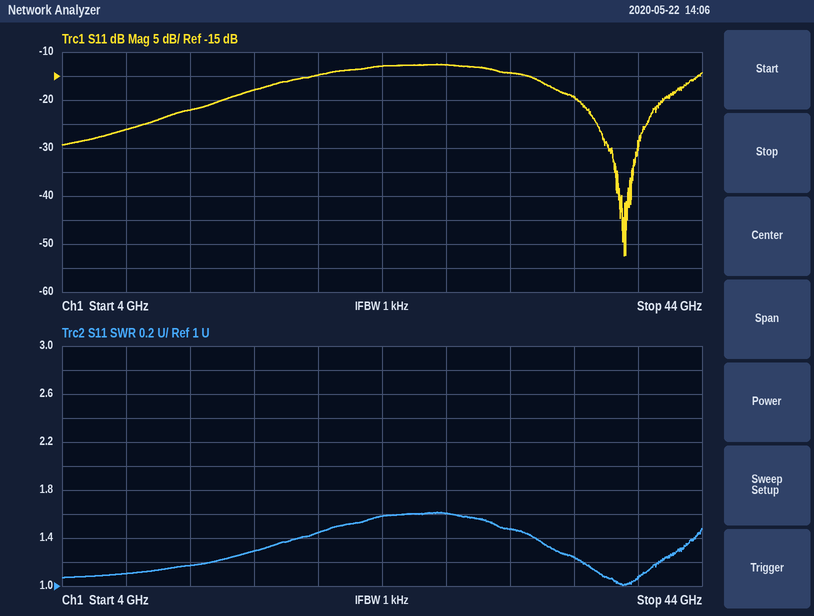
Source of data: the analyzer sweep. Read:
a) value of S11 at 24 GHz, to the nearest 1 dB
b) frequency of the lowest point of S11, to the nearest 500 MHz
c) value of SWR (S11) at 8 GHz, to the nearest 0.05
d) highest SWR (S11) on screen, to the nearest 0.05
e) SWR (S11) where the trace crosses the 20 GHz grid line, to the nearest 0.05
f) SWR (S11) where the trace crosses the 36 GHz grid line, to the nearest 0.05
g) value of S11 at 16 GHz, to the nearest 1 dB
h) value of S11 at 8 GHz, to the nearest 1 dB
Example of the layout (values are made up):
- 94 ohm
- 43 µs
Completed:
- -13 dB
- 39.0 GHz
- 1.10
- 1.60
- 1.45
- 1.25
- -18 dB
- -26 dB
